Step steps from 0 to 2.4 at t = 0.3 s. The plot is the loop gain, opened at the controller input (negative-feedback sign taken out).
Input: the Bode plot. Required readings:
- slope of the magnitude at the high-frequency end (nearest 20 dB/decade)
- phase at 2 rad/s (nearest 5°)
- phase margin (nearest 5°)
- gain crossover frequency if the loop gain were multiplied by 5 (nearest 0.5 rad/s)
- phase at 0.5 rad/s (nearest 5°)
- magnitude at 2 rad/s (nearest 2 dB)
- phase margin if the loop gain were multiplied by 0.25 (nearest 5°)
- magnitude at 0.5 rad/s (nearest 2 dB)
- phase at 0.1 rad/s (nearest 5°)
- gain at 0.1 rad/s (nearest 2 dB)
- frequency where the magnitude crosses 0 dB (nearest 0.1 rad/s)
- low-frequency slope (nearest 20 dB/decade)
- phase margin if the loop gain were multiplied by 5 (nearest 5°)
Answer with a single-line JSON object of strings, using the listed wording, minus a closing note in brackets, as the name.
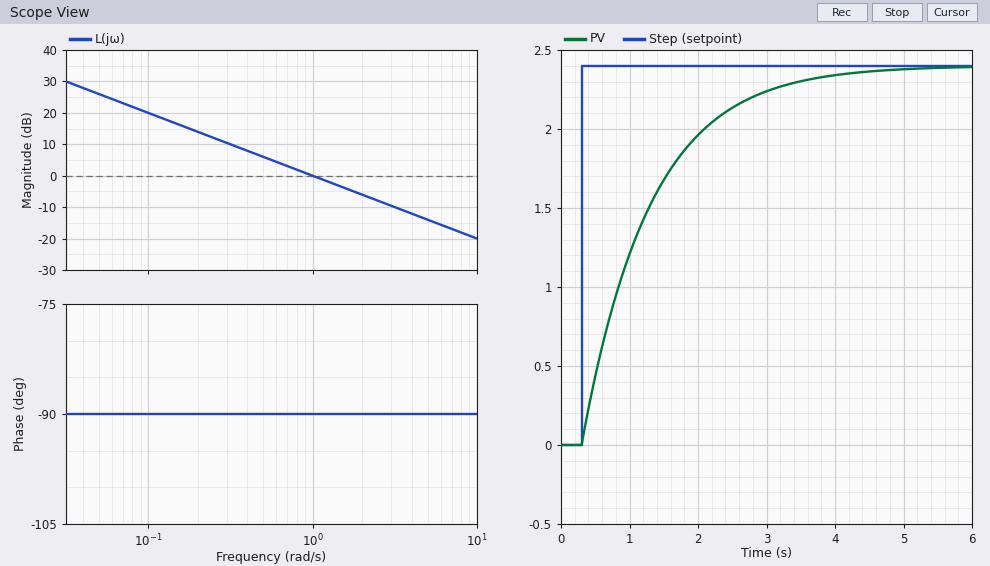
{"slope of the magnitude at the high-frequency end": "-20 dB/decade", "phase at 2 rad/s": "-90°", "phase margin": "90°", "gain crossover frequency if the loop gain were multiplied by 5": "5.0 rad/s", "phase at 0.5 rad/s": "-90°", "magnitude at 2 rad/s": "-6 dB", "phase margin if the loop gain were multiplied by 0.25": "90°", "magnitude at 0.5 rad/s": "6 dB", "phase at 0.1 rad/s": "-90°", "gain at 0.1 rad/s": "20 dB", "frequency where the magnitude crosses 0 dB": "1.0 rad/s", "low-frequency slope": "-20 dB/decade", "phase margin if the loop gain were multiplied by 5": "90°"}
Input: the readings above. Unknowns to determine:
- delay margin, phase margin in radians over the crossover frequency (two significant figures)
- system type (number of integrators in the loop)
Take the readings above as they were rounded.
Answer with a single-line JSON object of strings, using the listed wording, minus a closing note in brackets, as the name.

{"delay margin, phase margin in radians over the crossover frequency": "1.6 s", "system type": "1"}
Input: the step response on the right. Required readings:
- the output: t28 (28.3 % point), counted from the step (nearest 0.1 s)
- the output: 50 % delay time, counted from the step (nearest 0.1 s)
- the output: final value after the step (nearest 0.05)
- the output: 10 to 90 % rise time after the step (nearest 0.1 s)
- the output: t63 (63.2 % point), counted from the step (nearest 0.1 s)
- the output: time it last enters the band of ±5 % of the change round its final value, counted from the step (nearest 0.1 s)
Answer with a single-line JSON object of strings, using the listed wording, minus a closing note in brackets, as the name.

{"the output: t28 (28.3 % point), counted from the step": "0.3 s", "the output: 50 % delay time, counted from the step": "0.7 s", "the output: final value after the step": "2.40", "the output: 10 to 90 % rise time after the step": "2.2 s", "the output: t63 (63.2 % point), counted from the step": "1.0 s", "the output: time it last enters the band of ±5 % of the change round its final value, counted from the step": "3.0 s"}
